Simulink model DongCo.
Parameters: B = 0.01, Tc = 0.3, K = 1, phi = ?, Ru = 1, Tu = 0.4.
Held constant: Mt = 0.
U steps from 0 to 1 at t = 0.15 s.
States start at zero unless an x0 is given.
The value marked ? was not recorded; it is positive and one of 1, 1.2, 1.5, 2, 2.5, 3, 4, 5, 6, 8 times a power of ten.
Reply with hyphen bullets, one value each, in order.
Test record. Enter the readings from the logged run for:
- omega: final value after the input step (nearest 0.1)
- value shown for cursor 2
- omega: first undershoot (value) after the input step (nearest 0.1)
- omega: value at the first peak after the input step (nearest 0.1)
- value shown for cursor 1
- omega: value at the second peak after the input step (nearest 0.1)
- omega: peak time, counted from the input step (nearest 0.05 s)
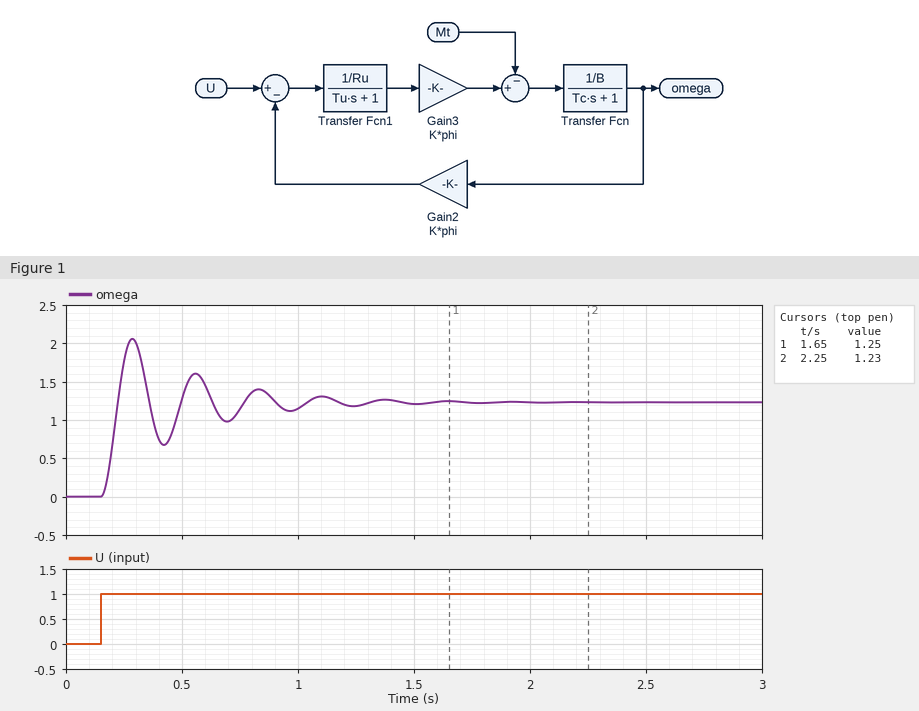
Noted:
- 1.2
- 1.23
- 0.7
- 2.1
- 1.25
- 1.6
- 0.15 s
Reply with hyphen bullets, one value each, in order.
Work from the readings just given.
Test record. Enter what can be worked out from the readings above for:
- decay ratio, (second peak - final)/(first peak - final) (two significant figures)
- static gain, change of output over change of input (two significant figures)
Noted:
- 0.44
- 1.2
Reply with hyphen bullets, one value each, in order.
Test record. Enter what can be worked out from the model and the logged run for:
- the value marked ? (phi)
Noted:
- 0.8
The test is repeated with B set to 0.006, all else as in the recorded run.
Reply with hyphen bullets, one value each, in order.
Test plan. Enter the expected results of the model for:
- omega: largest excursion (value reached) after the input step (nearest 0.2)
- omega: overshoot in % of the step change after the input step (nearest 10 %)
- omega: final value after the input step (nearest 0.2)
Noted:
- 2.2
- 70 %
- 1.2
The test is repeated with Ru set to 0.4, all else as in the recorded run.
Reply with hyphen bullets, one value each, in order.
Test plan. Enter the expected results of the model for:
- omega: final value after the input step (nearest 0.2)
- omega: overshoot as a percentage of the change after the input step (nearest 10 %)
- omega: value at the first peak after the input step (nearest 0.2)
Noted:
- 1.2
- 80 %
- 2.2
